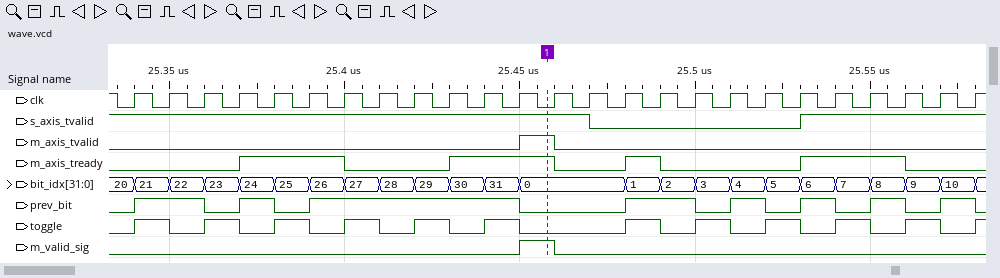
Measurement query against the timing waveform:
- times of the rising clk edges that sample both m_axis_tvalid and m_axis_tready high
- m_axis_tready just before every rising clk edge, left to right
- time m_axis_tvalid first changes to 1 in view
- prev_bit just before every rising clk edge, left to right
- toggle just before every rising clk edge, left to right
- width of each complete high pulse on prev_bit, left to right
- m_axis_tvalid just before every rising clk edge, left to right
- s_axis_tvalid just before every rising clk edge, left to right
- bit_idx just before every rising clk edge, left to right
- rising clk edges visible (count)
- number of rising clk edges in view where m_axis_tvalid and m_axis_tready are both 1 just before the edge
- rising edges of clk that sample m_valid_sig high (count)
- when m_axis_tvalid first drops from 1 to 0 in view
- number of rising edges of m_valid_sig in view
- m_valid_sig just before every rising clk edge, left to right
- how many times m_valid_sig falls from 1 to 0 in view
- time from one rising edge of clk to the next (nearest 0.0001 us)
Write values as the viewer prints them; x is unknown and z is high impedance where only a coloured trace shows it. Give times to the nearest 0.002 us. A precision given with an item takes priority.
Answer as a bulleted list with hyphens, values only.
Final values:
- 25.46 us
- 0 0 0 0 1 1 1 0 0 0 1 1 1 0 0 1 0 0 0 0 1 1 1 0 0
- 25.45 us
- 0 1 1 0 1 0 1 1 1 1 1 1 0 0 0 1 1 0 1 0 1 0 1 0 1
- 0 1 0 1 0 1 0 1 0 1 0 1 0 0 0 1 0 1 0 1 0 1 0 1 0
- 0.02 us, 0.01 us, 0.06 us, 0.02 us, 0.01 us, 0.01 us, 0.01 us, 0.01 us
- 0 0 0 0 0 0 0 0 0 0 0 0 1 0 0 0 0 0 0 0 0 0 0 0 0
- 1 1 1 1 1 1 1 1 1 1 1 1 1 1 0 0 0 0 0 0 1 1 1 1 1
- 20, 21, 22, 23, 24, 25, 26, 27, 28, 29, 30, 31, 0, 0, 0, 1, 2, 3, 4, 5, 6, 7, 8, 9, 10
- 25
- 1
- 1
- 25.46 us
- 1
- 0 0 0 0 0 0 0 0 0 0 0 0 1 0 0 0 0 0 0 0 0 0 0 0 0
- 1
- 0.01 us
